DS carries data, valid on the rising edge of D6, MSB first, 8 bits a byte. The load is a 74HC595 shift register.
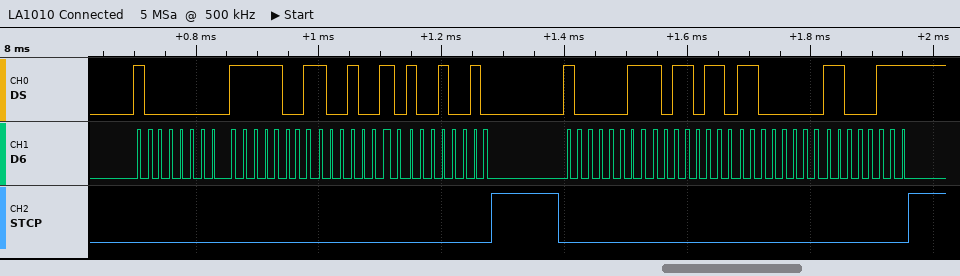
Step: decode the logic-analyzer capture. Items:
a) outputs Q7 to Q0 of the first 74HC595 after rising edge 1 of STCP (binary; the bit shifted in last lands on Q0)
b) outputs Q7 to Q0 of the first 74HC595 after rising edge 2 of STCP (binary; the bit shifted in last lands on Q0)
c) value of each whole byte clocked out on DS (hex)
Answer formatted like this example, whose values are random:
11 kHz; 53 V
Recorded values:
10010010; 11000111; 80 F9 92 92 83 B6 C0 C7
